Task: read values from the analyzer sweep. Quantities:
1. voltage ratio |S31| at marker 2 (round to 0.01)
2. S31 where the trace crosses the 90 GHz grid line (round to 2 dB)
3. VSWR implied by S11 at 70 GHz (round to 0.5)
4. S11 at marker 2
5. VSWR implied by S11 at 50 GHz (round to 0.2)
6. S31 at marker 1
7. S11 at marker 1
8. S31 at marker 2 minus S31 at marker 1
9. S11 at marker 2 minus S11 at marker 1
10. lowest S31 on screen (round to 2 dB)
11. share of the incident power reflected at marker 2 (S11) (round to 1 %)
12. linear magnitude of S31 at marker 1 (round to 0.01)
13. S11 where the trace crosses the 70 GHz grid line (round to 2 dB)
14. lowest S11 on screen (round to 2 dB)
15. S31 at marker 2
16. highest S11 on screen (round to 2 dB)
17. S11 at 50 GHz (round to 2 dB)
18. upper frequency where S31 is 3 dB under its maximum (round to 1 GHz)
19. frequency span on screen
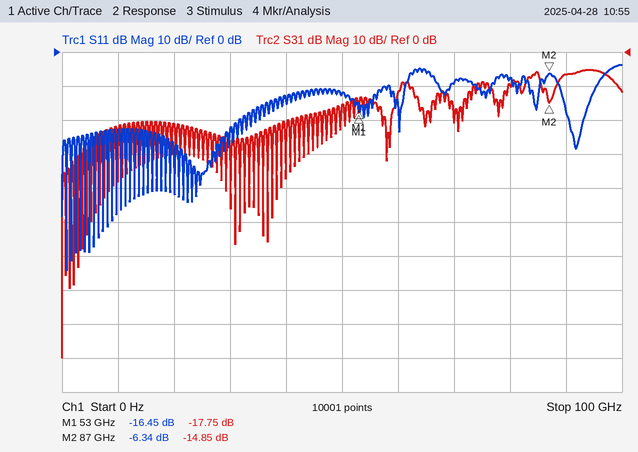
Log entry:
0.18
-6 dB
2.0
-6.34 dB
1.6
-17.75 dB
-16.45 dB
2.90 dB
10.11 dB
-90 dB
23 %
0.13
-10 dB
-64 dB
-14.85 dB
-4 dB
-12 dB
98 GHz
100 GHz
